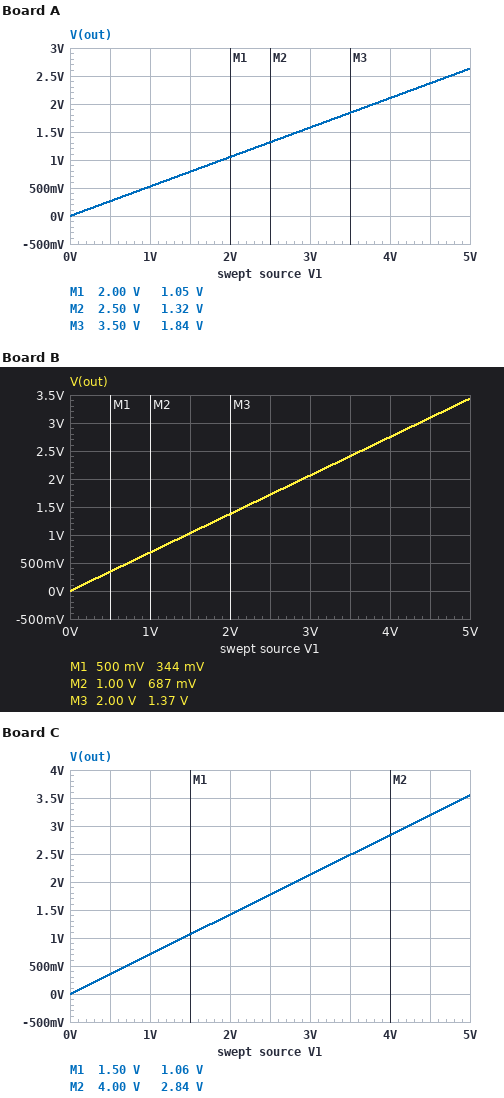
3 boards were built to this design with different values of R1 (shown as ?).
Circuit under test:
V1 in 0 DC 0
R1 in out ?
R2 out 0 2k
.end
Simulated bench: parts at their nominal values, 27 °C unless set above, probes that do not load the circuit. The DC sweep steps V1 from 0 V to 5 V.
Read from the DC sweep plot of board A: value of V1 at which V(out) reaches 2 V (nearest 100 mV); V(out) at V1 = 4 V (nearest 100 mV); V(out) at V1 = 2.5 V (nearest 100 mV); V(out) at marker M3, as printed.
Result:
3.8 V
2.1 V
1.3 V
1.84 V
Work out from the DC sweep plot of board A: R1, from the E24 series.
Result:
1.8 kΩ
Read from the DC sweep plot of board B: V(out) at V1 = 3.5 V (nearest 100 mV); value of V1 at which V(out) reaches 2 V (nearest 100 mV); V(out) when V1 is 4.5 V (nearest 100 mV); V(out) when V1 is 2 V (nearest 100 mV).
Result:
2.4 V
2.9 V
3.1 V
1.4 V
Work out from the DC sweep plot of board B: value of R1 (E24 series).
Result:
910 Ω
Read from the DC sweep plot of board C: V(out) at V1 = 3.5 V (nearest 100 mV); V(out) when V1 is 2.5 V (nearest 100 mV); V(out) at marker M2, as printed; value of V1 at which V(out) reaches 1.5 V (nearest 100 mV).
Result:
2.5 V
1.8 V
2.84 V
2.1 V
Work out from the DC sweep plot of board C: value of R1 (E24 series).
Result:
820 Ω
